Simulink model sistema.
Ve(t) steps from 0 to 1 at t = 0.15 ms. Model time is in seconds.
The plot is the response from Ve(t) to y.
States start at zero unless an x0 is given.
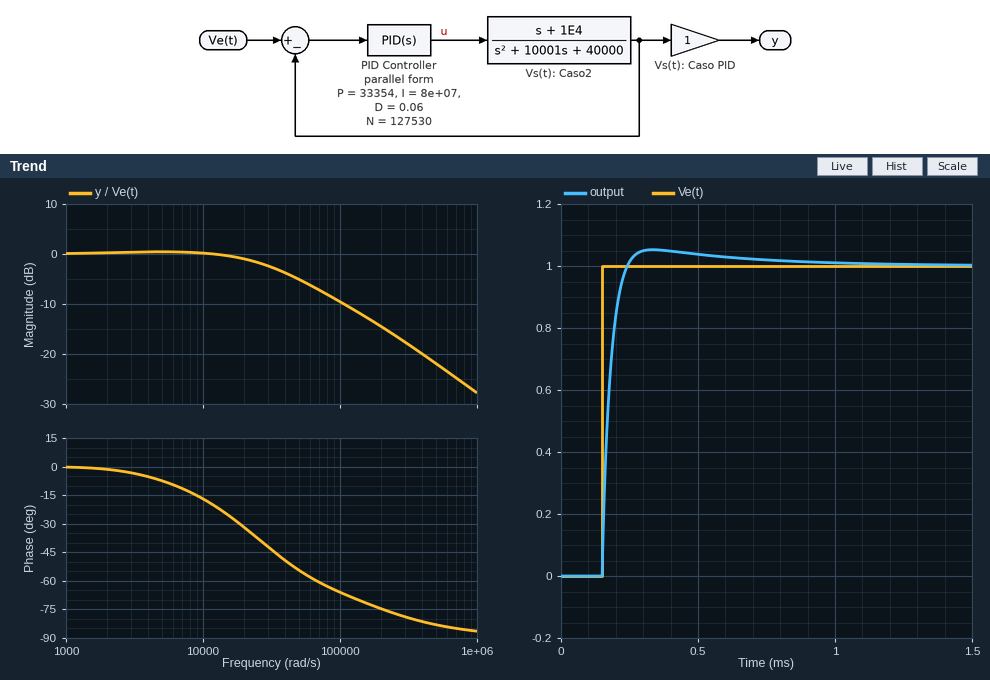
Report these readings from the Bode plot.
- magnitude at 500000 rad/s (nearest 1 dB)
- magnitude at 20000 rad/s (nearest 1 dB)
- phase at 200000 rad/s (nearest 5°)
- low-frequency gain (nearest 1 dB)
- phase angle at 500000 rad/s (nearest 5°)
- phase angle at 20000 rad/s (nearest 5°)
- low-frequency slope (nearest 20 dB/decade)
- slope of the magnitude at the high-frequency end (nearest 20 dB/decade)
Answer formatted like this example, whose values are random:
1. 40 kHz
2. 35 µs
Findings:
1. -22 dB
2. -1 dB
3. -75°
4. 0 dB
5. -85°
6. -30°
7. 0 dB/decade
8. -20 dB/decade
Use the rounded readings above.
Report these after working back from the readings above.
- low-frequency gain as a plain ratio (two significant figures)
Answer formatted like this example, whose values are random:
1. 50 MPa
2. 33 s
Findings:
1. 1.0
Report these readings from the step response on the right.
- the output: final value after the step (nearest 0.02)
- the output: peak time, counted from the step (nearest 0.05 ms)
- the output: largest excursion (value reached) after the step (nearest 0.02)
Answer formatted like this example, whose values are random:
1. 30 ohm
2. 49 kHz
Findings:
1. 1.00
2. 0.20 ms
3. 1.06
